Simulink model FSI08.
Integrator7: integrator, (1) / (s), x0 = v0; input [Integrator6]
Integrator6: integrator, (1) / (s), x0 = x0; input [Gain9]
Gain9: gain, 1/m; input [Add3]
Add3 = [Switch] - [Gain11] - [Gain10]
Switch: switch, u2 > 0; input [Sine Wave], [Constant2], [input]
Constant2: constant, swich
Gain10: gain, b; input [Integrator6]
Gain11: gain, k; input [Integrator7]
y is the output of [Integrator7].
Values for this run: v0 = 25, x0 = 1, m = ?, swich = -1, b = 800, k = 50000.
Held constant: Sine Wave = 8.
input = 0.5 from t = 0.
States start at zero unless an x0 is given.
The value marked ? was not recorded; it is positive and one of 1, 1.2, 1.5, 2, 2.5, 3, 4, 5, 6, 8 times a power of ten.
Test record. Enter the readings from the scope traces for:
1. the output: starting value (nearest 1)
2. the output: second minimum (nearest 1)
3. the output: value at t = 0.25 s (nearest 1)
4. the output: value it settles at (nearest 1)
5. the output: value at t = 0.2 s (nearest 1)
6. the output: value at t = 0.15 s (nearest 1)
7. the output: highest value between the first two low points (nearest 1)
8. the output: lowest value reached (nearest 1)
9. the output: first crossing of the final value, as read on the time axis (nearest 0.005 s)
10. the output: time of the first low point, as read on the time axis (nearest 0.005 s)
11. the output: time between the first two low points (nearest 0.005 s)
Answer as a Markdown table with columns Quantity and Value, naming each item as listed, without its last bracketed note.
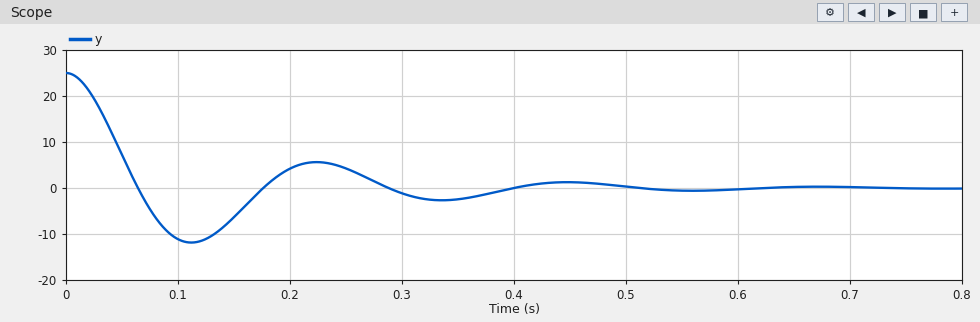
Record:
| Quantity | Value |
|---|---|
| the output: starting value | 25 |
| the output: second minimum | -3 |
| the output: value at t = 0.25 s | 4 |
| the output: value it settles at | 0 |
| the output: value at t = 0.2 s | 4 |
| the output: value at t = 0.15 s | -6 |
| the output: highest value between the first two low points | 6 |
| the output: lowest value reached | -12 |
| the output: first crossing of the final value, as read on the time axis | 0.065 s |
| the output: time of the first low point, as read on the time axis | 0.110 s |
| the output: time between the first two low points | 0.225 s |
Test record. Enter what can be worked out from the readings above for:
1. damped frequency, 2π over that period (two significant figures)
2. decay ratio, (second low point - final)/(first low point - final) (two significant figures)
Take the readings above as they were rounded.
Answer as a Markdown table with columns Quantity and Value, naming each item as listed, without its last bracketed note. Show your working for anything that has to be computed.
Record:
| Quantity | Value |
|---|---|
| damped frequency, 2π over that period | 2π / 0.225 = 28 rad/s |
| decay ratio, (second low point - final)/(first low point - final) | (-3 - 0) / (-12 - 0) = 0.25 |
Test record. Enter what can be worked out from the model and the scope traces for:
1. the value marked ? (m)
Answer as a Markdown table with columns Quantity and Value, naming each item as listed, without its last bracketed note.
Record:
| Quantity | Value |
|---|---|
| the value marked ? | 60 |
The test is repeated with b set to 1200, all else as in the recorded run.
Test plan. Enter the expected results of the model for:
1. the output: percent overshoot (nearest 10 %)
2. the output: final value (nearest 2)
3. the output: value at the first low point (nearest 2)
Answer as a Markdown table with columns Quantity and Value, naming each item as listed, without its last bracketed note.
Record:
| Quantity | Value |
|---|---|
| the output: percent overshoot | 30 % |
| the output: final value | 0 |
| the output: value at the first low point | -8 |
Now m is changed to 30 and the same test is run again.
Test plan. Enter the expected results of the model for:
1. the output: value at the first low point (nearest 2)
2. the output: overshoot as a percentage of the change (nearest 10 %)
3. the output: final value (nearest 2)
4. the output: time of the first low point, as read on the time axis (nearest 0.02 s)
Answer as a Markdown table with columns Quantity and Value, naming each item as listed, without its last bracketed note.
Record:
| Quantity | Value |
|---|---|
| the output: value at the first low point | -8 |
| the output: overshoot as a percentage of the change | 30 % |
| the output: final value | 0 |
| the output: time of the first low point, as read on the time axis | 0.08 s |
